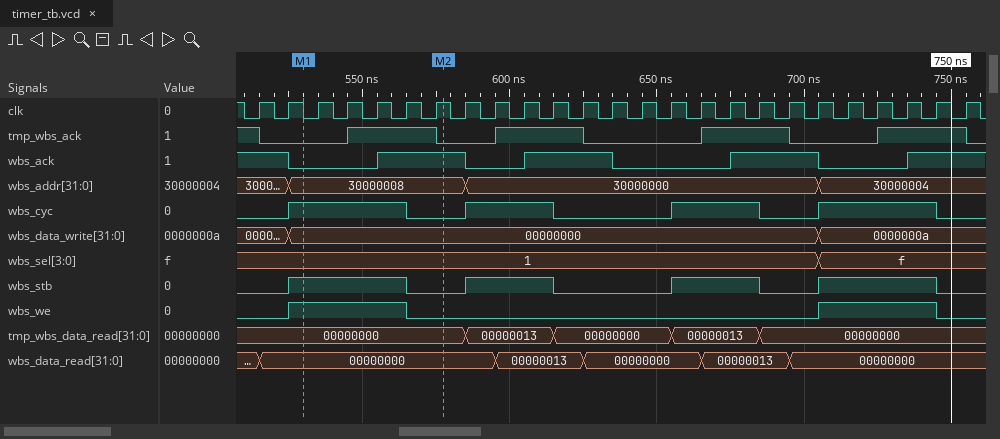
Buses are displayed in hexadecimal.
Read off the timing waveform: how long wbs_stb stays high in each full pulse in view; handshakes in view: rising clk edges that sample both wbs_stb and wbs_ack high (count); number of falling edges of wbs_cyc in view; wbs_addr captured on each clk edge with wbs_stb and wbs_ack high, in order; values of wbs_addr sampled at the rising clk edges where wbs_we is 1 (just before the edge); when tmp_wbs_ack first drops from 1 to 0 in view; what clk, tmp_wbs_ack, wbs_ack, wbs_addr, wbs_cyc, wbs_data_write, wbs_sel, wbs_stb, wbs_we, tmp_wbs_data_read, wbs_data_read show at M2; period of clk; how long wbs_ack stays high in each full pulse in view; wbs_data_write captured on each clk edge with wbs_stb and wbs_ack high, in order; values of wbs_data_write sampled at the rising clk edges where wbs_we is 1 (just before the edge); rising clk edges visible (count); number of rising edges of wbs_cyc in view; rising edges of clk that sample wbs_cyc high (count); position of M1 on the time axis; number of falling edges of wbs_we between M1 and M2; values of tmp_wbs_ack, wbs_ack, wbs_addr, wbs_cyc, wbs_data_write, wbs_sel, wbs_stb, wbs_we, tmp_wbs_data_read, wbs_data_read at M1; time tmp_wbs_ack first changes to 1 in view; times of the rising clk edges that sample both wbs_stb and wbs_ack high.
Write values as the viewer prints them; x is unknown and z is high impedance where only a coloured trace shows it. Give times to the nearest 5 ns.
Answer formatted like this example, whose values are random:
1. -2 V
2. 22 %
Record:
1. 40 ns, 30 ns, 30 ns, 40 ns
2. 4
3. 4
4. 30000008, 30000000, 30000000, 30000004
5. 30000008, 30000008, 30000008, 30000008, 30000004, 30000004, 30000004, 30000004
6. 515 ns
7. clk=1, tmp_wbs_ack=0, wbs_ack=1, wbs_addr=30000008, wbs_cyc=0, wbs_data_write=00000000, wbs_sel=1, wbs_stb=0, wbs_we=0, tmp_wbs_data_read=00000000, wbs_data_read=00000000
8. 10 ns
9. 30 ns, 30 ns, 30 ns
10. 00000000, 00000000, 00000000, 0000000a
11. 00000000, 00000000, 00000000, 00000000, 0000000a, 0000000a, 0000000a, 0000000a
12. 25
13. 4
14. 14
15. 530 ns
16. 1
17. tmp_wbs_ack=0, wbs_ack=0, wbs_addr=30000008, wbs_cyc=1, wbs_data_write=00000000, wbs_sel=1, wbs_stb=1, wbs_we=1, tmp_wbs_data_read=00000000, wbs_data_read=00000000
18. 545 ns
19. 565 ns, 615 ns, 685 ns, 745 ns
